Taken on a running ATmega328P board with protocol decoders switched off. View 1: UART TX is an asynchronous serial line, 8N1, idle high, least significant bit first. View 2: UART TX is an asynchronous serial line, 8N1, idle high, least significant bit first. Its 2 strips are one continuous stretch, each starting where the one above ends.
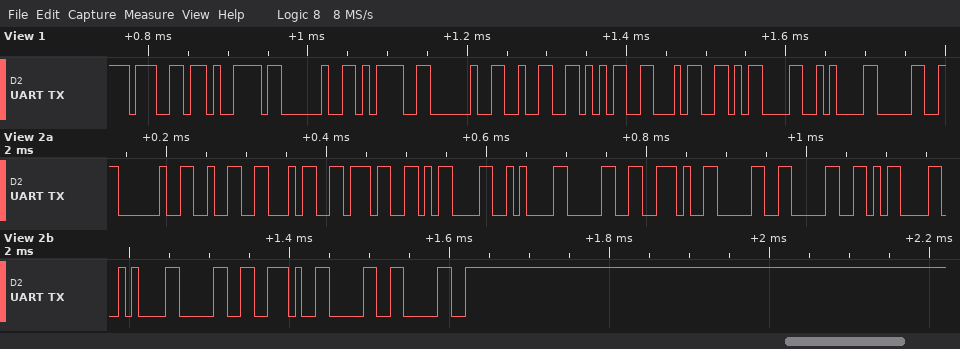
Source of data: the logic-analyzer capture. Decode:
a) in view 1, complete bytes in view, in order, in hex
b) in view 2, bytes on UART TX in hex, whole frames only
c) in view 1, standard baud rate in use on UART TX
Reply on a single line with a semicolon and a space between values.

67 79 20 3D 20 32 35 34 0D 0A 30; 20 32 34 37 0D 0A 30 2E 30 30 0D 0A 30 2E 30 30; 115200 baud
